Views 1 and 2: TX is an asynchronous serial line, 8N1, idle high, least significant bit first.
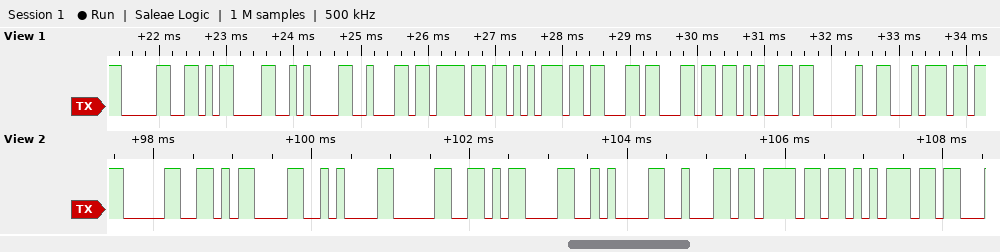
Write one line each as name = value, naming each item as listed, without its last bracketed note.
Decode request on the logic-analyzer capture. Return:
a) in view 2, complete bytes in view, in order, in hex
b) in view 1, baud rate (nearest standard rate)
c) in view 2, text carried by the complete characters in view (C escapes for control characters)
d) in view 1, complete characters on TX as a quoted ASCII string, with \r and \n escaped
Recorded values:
in view 2, complete bytes in view, in order, in hex = 0x30 0x0D 0x0A 0x30 0x0D 0x0A 0x62 0x6F 0x75
in view 1, baud rate = 9600 baud
in view 2, text carried by the complete characters in view = "0\r\n0\r\nbou"
in view 1, complete characters on TX as a quoted ASCII string, with \r and \n escaped = "0\r\nboucle t"
